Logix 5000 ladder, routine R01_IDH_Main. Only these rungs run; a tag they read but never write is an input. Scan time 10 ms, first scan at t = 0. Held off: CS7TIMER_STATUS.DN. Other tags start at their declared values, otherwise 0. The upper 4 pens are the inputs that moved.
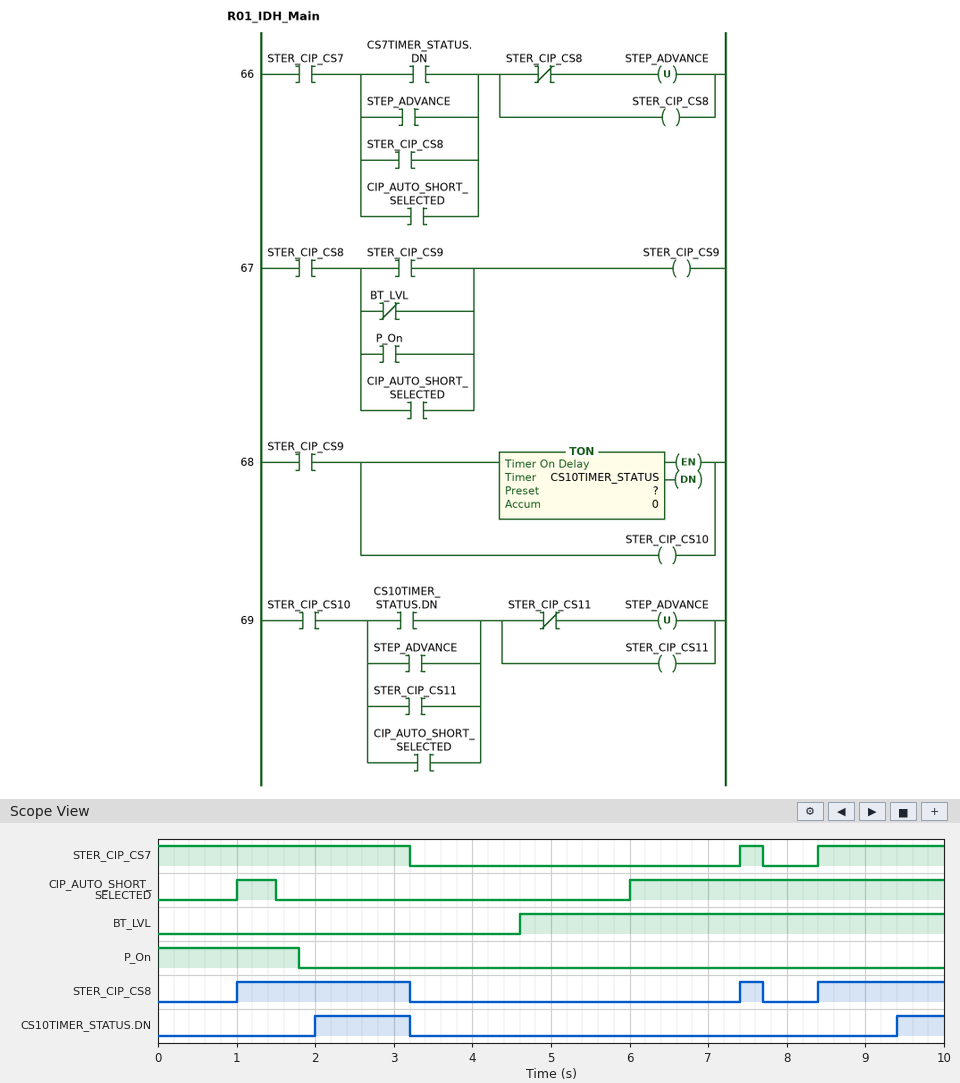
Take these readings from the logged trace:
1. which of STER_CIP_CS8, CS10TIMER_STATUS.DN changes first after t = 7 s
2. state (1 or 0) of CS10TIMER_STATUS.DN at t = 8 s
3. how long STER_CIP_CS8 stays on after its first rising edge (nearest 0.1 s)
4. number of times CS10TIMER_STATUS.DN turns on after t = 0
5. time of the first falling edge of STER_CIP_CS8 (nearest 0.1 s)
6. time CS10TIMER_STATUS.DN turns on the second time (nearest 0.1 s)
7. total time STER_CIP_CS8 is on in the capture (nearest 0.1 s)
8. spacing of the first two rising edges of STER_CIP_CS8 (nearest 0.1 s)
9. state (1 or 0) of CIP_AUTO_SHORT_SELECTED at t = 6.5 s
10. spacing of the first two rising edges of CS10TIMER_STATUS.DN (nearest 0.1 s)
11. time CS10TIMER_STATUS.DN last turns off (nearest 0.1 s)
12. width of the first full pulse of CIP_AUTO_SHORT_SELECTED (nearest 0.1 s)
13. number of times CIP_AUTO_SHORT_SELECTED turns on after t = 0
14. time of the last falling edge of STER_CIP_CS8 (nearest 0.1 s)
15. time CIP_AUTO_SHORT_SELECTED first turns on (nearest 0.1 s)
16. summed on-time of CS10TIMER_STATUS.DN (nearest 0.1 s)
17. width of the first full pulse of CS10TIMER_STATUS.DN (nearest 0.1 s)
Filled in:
STER_CIP_CS8
0
2.2 s
2
3.2 s
9.4 s
4.1 s
6.4 s
1
7.4 s
3.2 s
0.5 s
2
7.7 s
1.0 s
1.8 s
1.2 s
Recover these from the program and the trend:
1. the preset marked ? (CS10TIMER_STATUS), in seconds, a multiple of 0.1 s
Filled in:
1.0 s
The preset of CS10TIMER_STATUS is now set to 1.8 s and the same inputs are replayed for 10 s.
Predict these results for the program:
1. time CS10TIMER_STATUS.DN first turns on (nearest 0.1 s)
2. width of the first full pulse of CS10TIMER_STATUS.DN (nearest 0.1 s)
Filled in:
2.8 s
0.4 s
